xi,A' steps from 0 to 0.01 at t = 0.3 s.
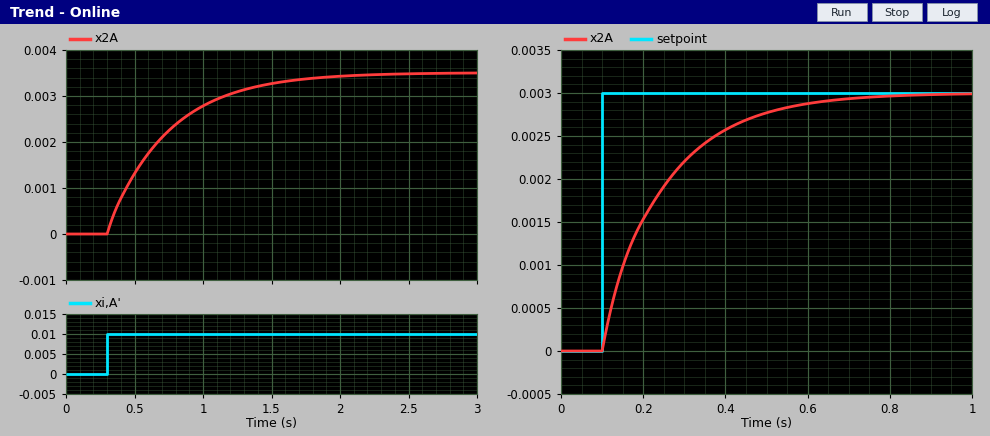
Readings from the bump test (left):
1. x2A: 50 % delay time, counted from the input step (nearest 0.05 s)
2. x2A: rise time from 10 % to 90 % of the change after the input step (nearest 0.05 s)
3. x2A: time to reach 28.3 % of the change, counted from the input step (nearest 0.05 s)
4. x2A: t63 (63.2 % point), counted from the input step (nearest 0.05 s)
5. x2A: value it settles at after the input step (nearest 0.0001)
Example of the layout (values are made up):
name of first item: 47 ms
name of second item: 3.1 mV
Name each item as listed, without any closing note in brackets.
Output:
x2A: 50 % delay time, counted from the input step: 0.30 s
x2A: rise time from 10 % to 90 % of the change after the input step: 1.00 s
x2A: time to reach 28.3 % of the change, counted from the input step: 0.15 s
x2A: t63 (63.2 % point), counted from the input step: 0.45 s
x2A: value it settles at after the input step: 0.0035
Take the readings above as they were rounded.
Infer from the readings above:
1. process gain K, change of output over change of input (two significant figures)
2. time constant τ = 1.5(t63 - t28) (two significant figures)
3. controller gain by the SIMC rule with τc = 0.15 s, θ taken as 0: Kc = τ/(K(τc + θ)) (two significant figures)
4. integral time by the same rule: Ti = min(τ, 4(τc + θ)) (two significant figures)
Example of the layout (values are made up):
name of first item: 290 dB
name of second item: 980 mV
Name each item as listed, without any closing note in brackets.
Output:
process gain K, change of output over change of input: 0.35
time constant τ = 1.5(t63 - t28): 0.45 s
controller gain by the SIMC rule with τc = 0.15 s, θ taken as 0: Kc = τ/(K(τc + θ)): 8.6
integral time by the same rule: Ti = min(τ, 4(τc + θ)): 0.45 s
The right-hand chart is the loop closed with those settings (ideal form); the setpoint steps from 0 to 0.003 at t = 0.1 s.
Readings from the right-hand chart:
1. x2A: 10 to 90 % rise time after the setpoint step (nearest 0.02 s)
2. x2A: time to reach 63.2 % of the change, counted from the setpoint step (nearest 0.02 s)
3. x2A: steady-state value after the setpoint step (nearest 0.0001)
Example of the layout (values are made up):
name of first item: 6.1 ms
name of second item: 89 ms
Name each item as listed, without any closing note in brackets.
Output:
x2A: 10 to 90 % rise time after the setpoint step: 0.34 s
x2A: time to reach 63.2 % of the change, counted from the setpoint step: 0.14 s
x2A: steady-state value after the setpoint step: 0.0030
